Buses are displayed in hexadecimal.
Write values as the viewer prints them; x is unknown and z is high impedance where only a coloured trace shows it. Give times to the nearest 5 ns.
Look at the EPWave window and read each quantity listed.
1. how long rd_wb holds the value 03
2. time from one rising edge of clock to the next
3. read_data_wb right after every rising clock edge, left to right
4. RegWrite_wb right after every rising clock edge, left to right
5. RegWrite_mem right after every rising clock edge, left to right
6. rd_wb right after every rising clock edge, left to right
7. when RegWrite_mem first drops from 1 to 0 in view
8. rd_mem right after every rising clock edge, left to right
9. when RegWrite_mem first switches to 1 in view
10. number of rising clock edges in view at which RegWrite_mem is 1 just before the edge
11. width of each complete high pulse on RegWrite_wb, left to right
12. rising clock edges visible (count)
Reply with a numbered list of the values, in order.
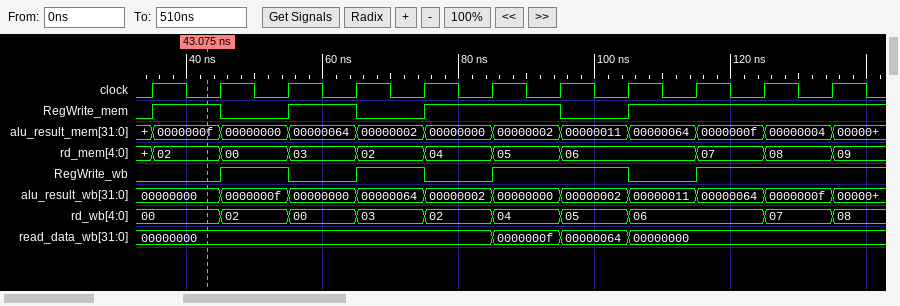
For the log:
1. 10 ns
2. 10 ns
3. 00000000, 00000000, 00000000, 00000000, 00000000, 0000000f, 00000064, 00000000, 00000000, 00000000, 00000000
4. 0 1 0 1 0 1 1 0 1 1 1
5. 1 0 1 0 1 1 0 1 1 1 1
6. 00, 02, 00, 03, 02, 04, 05, 06, 06, 07, 08
7. 45 ns
8. 02, 00, 03, 02, 04, 05, 06, 06, 07, 08, 09
9. 35 ns
10. 7
11. 10 ns, 10 ns, 20 ns
12. 11
